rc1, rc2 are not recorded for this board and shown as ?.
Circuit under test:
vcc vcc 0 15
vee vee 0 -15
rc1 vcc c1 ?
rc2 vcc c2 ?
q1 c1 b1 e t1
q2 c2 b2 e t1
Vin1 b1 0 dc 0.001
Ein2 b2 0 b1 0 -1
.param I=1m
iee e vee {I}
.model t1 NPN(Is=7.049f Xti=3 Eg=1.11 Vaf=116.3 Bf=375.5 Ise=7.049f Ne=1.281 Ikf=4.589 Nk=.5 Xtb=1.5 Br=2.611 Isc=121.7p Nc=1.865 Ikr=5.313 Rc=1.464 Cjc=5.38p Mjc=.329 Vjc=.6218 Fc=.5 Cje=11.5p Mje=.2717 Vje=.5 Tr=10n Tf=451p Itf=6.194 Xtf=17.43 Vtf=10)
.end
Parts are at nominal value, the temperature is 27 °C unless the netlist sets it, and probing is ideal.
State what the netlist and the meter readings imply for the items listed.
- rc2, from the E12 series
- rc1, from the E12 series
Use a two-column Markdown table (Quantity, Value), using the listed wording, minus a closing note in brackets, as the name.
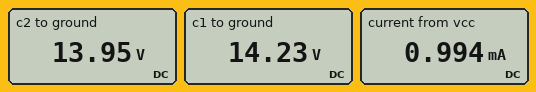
| Quantity | Value |
|---|---|
| rc2, from the E12 series | 2.2 kΩ |
| rc1, from the E12 series | 1.5 kΩ |
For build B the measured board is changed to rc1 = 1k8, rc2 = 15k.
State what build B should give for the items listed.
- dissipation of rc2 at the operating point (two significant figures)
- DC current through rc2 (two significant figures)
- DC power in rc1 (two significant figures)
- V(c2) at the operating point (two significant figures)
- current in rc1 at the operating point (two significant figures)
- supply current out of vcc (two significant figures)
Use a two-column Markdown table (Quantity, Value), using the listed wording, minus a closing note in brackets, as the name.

| Quantity | Value |
|---|---|
| dissipation of rc2 at the operating point | 3.3 mW |
| DC current through rc2 | 470 µA |
| DC power in rc1 | 500 µW |
| V(c2) at the operating point | 8.0 V |
| current in rc1 at the operating point | 530 µA |
| supply current out of vcc | 990 µA |
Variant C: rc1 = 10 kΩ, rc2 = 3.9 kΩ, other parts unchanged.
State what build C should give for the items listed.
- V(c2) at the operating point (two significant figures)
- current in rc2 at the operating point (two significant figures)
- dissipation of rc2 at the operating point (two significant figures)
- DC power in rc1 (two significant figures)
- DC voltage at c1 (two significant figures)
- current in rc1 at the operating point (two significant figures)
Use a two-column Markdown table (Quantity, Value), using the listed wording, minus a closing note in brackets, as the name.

| Quantity | Value |
|---|---|
| V(c2) at the operating point | 13 V |
| current in rc2 at the operating point | 480 µA |
| dissipation of rc2 at the operating point | 910 µW |
| DC power in rc1 | 2.6 mW |
| DC voltage at c1 | 9.9 V |
| current in rc1 at the operating point | 510 µA |
